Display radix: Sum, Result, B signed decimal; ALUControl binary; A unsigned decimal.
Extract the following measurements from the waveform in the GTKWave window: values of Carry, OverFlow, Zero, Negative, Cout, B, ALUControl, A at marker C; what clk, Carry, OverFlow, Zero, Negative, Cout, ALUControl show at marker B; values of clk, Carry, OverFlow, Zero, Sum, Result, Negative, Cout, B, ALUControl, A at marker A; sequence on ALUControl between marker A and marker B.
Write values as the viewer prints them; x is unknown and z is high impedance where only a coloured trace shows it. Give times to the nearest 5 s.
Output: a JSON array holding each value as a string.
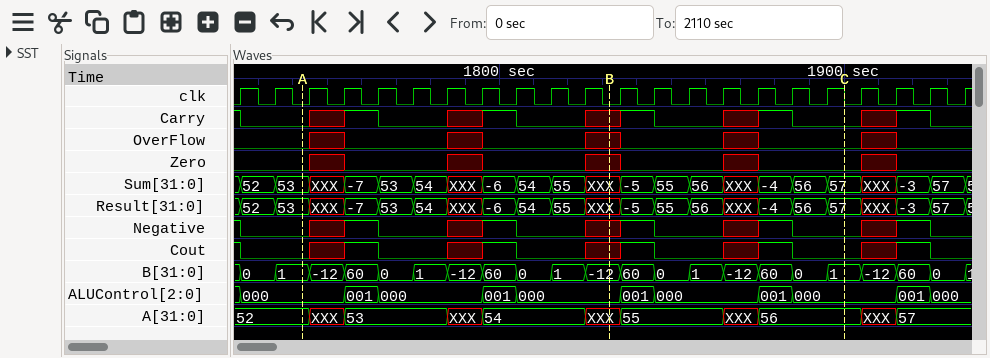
["Carry=0, OverFlow=0, Zero=0, Negative=0, Cout=0, B=1, ALUControl=000, A=56", "clk=0, Carry=x, OverFlow=x, Zero=x, Negative=x, Cout=x, ALUControl=000", "clk=0, Carry=0, OverFlow=0, Zero=0, Sum=53, Result=53, Negative=0, Cout=0, B=1, ALUControl=000, A=52", "000, 001, 000, 001, 000"]
